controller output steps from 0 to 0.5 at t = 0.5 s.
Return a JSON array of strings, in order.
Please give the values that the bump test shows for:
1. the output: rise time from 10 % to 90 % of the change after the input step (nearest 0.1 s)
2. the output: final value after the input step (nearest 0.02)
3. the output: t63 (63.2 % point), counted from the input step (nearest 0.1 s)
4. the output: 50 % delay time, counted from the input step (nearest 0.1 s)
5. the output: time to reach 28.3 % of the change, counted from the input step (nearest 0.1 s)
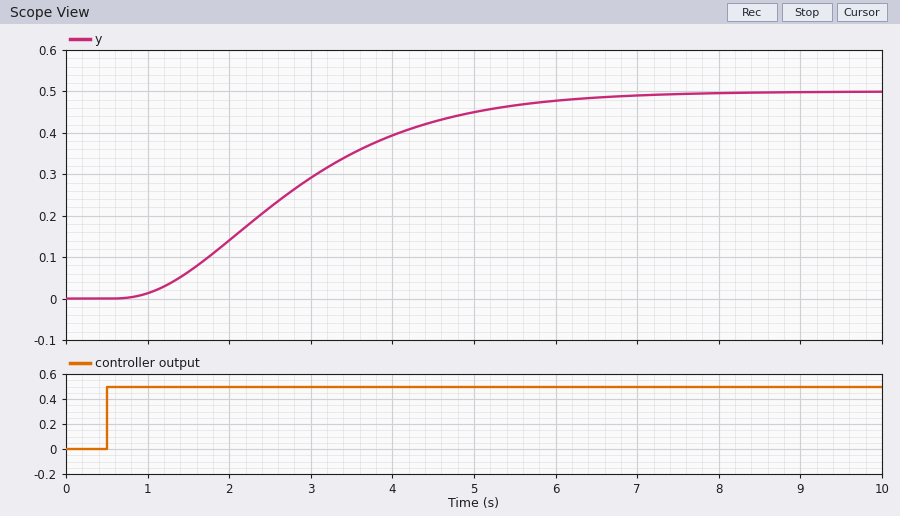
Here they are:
["3.6 s", "0.50", "2.7 s", "2.2 s", "1.5 s"]
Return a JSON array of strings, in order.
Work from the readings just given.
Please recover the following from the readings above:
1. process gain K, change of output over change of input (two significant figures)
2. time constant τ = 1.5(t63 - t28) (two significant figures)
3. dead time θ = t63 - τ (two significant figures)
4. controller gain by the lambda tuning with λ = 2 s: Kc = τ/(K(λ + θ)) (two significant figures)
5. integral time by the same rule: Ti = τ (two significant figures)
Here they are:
["1.0", "1.8 s", "0.90 s", "0.62", "1.8 s"]
